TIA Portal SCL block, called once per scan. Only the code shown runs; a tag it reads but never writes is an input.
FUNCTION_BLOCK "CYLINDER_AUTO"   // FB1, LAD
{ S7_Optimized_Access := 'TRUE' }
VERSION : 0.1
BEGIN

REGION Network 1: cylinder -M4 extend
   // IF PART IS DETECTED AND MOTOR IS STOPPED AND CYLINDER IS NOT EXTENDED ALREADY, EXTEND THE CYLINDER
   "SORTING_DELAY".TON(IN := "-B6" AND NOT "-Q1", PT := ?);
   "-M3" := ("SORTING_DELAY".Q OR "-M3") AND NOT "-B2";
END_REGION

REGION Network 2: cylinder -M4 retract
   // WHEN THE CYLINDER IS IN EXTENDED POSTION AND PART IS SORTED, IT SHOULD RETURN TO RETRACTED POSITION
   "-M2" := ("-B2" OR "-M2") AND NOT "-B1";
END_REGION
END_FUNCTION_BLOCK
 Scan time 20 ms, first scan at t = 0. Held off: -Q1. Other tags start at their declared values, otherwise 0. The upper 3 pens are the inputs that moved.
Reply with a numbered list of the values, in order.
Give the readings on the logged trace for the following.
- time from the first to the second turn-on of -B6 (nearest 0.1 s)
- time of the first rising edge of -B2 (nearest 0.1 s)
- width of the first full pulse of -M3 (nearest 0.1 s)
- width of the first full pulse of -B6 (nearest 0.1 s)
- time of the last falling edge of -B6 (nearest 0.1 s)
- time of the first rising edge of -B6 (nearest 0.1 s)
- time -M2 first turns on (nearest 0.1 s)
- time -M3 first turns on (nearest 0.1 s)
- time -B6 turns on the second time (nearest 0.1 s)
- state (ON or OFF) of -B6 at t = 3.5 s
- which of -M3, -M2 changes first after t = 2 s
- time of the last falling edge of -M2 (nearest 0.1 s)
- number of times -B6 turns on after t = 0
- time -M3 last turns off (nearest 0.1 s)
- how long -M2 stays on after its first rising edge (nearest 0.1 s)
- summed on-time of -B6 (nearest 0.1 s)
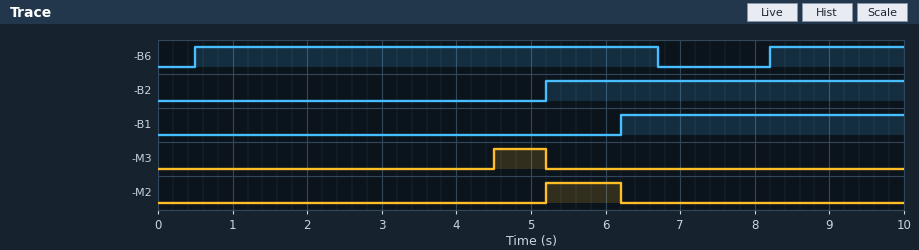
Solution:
1. 7.7 s
2. 5.2 s
3. 0.7 s
4. 6.2 s
5. 6.7 s
6. 0.5 s
7. 5.2 s
8. 4.5 s
9. 8.2 s
10. ON
11. -M3
12. 6.2 s
13. 2
14. 5.2 s
15. 1.0 s
16. 8.0 s
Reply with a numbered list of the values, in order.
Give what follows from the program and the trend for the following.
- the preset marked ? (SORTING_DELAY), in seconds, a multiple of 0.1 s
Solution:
1. 4.0 s
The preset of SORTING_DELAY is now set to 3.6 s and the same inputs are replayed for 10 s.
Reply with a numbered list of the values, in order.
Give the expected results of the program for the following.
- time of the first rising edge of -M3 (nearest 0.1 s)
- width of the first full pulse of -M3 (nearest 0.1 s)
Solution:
1. 4.1 s
2. 1.1 s
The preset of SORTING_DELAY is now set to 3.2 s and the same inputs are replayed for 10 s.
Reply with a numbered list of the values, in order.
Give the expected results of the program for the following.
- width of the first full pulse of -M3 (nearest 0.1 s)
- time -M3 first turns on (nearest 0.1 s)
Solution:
1. 1.5 s
2. 3.7 s
